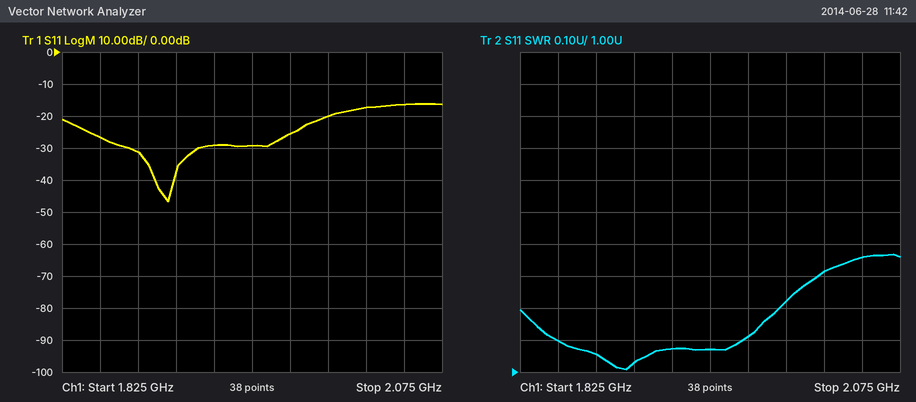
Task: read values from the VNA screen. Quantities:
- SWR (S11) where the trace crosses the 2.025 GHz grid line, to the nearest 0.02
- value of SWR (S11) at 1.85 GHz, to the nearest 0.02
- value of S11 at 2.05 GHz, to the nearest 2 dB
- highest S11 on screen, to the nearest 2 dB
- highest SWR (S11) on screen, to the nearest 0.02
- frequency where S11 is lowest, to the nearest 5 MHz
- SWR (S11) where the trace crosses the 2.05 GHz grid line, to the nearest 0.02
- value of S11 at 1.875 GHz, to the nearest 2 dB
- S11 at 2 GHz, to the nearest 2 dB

1.32
1.10
-16 dB
-16 dB
1.36
1.895 GHz
1.36
-32 dB
-20 dB
